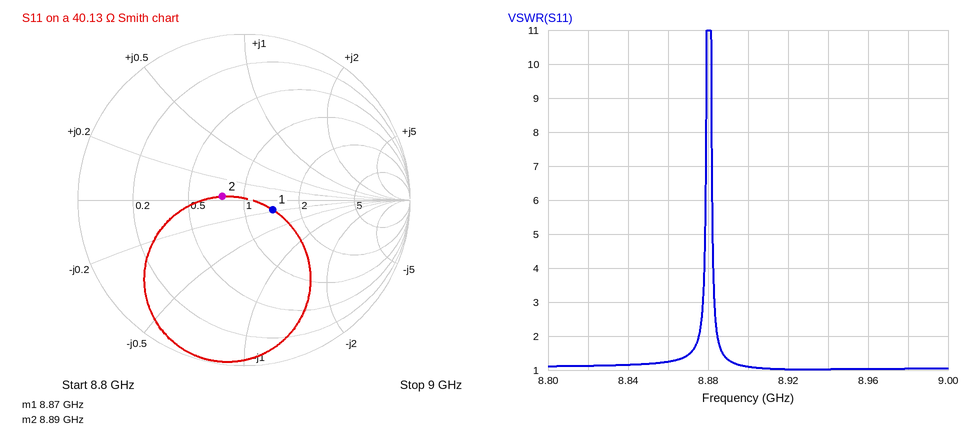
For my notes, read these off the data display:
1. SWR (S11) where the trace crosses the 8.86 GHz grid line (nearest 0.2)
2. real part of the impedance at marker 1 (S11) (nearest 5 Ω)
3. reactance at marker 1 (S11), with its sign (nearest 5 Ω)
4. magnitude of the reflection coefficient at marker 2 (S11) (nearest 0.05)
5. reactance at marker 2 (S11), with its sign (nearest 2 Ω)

1.2
55 Ω
-5 Ω
0.15
+2 Ω
